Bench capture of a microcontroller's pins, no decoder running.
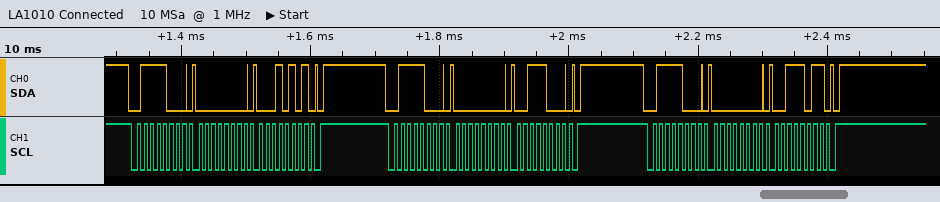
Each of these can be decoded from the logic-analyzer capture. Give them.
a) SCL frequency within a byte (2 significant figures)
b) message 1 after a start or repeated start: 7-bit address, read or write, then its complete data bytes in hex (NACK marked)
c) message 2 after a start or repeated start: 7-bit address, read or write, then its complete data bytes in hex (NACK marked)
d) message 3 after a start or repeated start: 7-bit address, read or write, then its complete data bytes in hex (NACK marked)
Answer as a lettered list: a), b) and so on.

a) 100 kHz
b) 0x3C write: 00 15
c) 0x3C write: 00 38
d) 0x3C write: 00 3B
